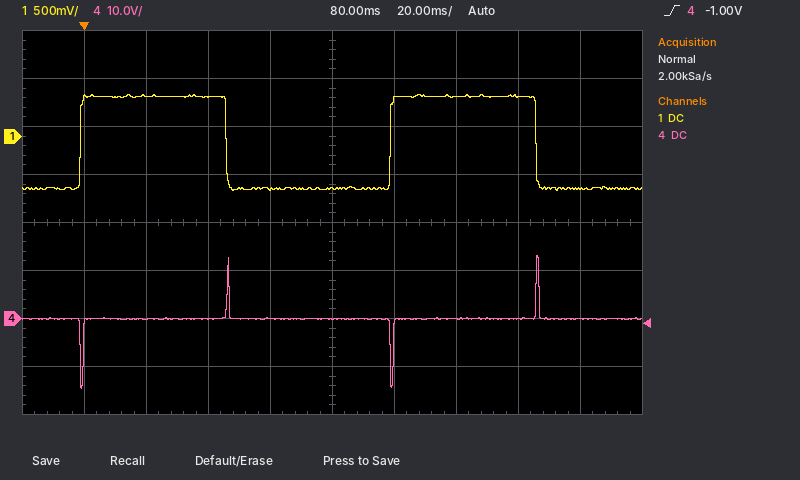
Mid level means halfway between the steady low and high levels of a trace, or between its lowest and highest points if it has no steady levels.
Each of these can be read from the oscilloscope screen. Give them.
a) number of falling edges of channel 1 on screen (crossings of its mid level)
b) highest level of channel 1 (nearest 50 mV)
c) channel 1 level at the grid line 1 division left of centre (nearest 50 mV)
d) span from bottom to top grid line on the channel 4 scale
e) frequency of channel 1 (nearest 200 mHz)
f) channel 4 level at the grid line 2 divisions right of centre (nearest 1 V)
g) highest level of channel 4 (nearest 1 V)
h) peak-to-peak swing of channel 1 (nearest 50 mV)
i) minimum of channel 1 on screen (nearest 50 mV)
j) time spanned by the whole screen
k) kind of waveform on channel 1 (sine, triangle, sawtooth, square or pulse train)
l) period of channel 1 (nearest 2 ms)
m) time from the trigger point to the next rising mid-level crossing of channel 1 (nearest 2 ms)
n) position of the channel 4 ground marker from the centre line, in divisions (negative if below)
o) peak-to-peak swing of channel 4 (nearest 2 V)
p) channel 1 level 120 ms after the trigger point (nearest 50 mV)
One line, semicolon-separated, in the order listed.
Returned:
2; 450 mV; -550 mV; 80 V; 10.0 Hz; 0 V; 13 V; 1.00 V; -550 mV; 200 ms; square; 100 ms; 98 ms; -2.0 div; 28 V; 400 mV
